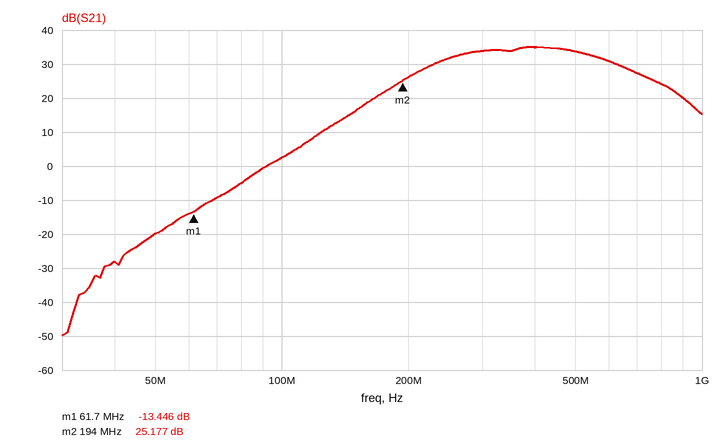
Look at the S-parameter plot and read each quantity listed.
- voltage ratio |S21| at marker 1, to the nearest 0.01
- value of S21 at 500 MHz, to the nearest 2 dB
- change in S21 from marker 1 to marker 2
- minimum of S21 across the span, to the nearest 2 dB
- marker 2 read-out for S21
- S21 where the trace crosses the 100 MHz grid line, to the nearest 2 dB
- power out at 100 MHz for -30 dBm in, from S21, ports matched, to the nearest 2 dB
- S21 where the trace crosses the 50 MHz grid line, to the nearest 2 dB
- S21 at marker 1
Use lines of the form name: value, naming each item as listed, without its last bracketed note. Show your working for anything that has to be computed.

voltage ratio |S21| at marker 1, to the nearest 0.01: 10^(-13.446/20) ≈ 0.21
value of S21 at 500 MHz, to the nearest 2 dB: 34 dB
change in S21 from marker 1 to marker 2: 25.177 − (-13.446) = 38.623 dB
minimum of S21 across the span, to the nearest 2 dB: -50 dB
marker 2 read-out for S21: 25.177 dB
S21 where the trace crosses the 100 MHz grid line, to the nearest 2 dB: 2 dB
power out at 100 MHz for -30 dBm in, from S21, ports matched, to the nearest 2 dB: -30 dBm + (2 dB) = -28 dBm
S21 where the trace crosses the 50 MHz grid line, to the nearest 2 dB: -20 dB
S21 at marker 1: -13.446 dB
